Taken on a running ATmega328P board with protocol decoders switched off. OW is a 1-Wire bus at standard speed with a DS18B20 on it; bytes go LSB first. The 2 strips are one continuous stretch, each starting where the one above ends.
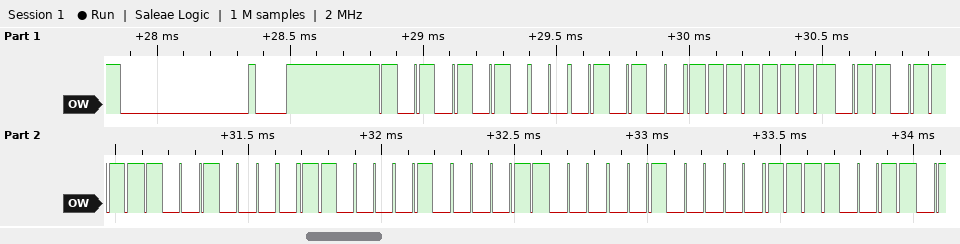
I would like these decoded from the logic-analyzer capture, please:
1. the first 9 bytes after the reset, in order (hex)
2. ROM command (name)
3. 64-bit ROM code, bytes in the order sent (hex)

55 28 FF F6 09 43 18 04 CF
Match ROM
28 FF F6 09 43 18 04 CF
